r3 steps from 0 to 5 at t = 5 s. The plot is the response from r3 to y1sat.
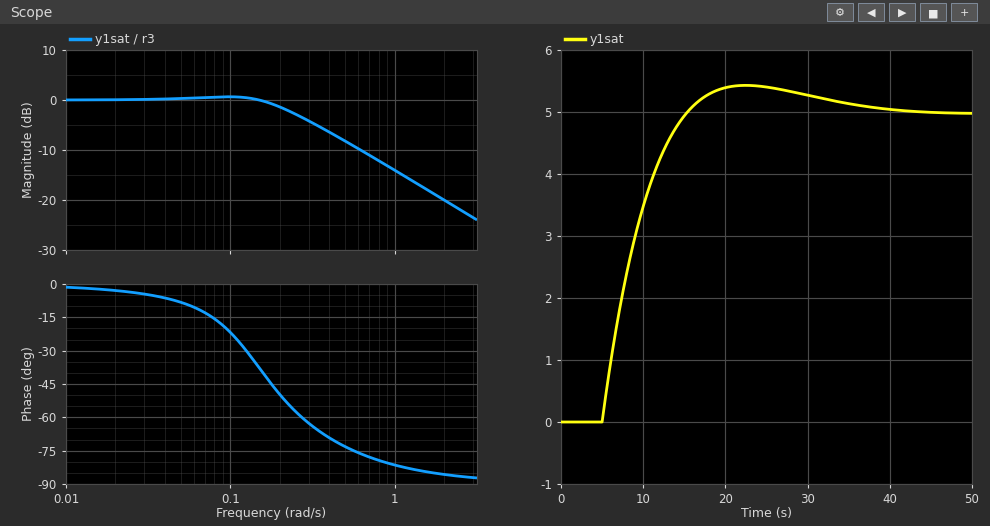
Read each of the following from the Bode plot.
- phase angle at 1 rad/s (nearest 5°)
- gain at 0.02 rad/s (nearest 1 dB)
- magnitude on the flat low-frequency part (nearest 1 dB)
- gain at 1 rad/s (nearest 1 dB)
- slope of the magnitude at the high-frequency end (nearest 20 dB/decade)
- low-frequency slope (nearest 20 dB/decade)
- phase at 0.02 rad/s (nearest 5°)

-80°
0 dB
0 dB
-14 dB
-20 dB/decade
0 dB/decade
-5°
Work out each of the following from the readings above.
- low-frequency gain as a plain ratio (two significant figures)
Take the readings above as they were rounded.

1.0
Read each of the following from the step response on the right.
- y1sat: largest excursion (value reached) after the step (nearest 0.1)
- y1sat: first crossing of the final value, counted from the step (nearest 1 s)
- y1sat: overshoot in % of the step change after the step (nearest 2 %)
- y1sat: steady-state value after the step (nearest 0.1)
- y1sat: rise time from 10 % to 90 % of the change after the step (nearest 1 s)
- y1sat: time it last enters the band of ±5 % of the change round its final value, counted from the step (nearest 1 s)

5.4
10 s
8 %
5.0
7 s
26 s
